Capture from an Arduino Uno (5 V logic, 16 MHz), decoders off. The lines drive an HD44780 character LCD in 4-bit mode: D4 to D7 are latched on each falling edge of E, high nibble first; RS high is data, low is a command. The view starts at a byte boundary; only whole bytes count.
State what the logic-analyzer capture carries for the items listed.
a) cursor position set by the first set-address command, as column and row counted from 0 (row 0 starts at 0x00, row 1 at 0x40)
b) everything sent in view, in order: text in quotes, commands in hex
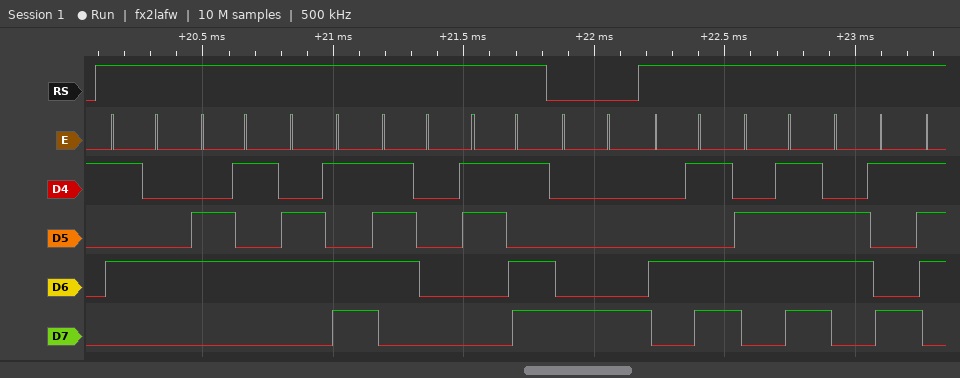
column 8, row 0
"Temp=" 0x88 "Moi"
